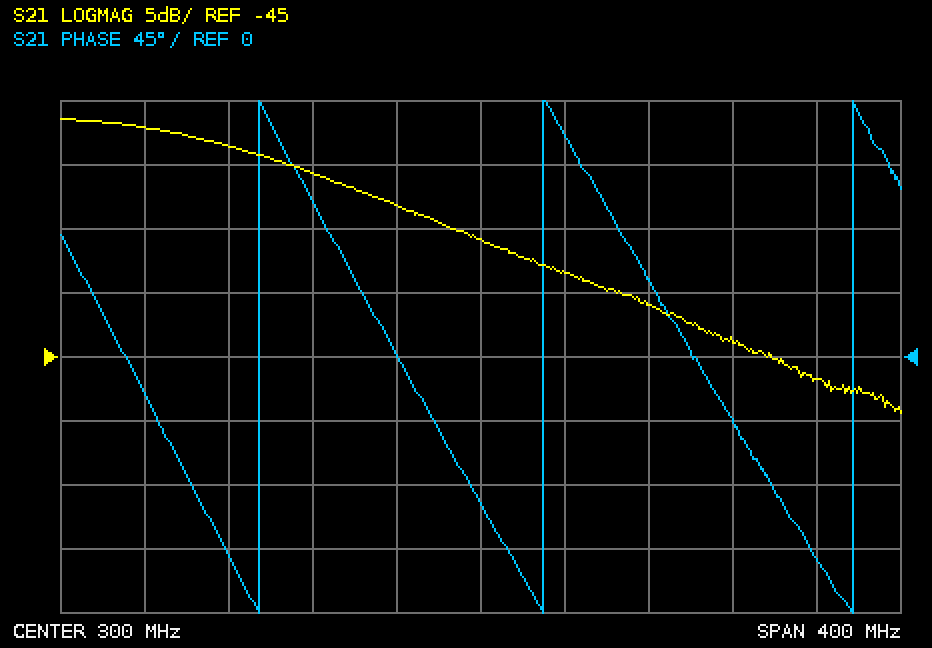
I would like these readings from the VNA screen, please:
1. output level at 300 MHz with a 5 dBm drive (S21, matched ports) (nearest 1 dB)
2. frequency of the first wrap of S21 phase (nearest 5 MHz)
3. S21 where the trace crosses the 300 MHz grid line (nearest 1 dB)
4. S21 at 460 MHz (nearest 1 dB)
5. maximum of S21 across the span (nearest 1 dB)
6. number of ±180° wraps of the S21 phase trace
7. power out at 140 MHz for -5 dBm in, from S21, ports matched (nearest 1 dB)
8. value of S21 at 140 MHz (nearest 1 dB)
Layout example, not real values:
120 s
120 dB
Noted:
-31 dBm
195 MHz
-36 dB
-47 dB
-26 dB
3
-32 dBm
-27 dB
